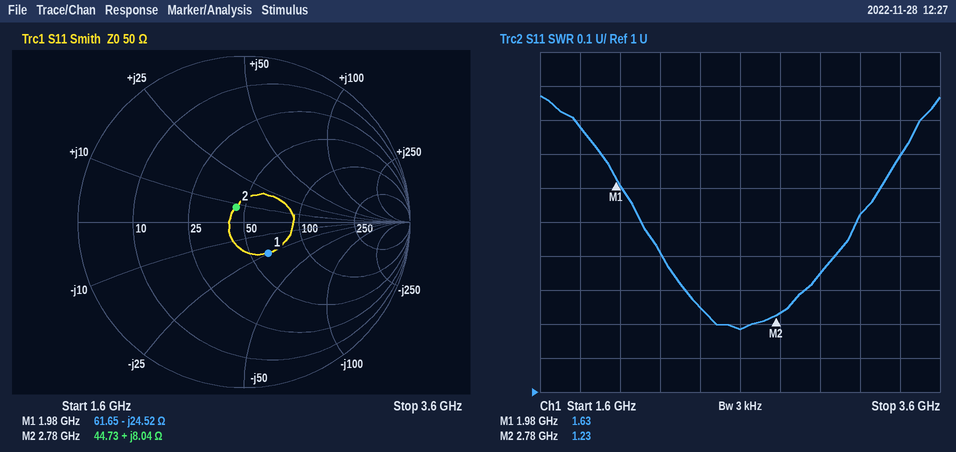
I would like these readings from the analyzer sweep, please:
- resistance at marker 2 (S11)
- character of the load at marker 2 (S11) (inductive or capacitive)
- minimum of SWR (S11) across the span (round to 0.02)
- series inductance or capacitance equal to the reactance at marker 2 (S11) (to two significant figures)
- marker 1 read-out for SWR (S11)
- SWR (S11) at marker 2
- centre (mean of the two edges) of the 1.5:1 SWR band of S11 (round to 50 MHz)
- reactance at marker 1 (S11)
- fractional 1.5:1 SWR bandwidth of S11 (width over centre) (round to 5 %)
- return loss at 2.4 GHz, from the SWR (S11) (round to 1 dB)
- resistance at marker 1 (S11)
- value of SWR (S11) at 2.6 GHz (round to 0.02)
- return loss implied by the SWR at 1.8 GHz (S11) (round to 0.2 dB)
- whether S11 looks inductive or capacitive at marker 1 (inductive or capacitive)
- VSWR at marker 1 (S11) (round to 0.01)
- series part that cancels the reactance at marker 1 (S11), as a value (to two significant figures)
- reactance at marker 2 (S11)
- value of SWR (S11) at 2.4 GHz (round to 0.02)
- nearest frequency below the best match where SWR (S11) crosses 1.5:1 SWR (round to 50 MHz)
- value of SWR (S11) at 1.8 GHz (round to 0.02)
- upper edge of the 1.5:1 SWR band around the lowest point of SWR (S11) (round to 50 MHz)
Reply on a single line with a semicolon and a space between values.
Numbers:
44.73 Ω; inductive; 1.18; 460 pH; 1.63; 1.23; 2.65 GHz; -24.52 Ω; 40 %; 19 dB; 61.65 Ω; 1.18; 11.0 dB; capacitive; 1.62; 2.0 nH; +8.04 Ω; 1.24; 2.10 GHz; 1.78; 3.20 GHz
